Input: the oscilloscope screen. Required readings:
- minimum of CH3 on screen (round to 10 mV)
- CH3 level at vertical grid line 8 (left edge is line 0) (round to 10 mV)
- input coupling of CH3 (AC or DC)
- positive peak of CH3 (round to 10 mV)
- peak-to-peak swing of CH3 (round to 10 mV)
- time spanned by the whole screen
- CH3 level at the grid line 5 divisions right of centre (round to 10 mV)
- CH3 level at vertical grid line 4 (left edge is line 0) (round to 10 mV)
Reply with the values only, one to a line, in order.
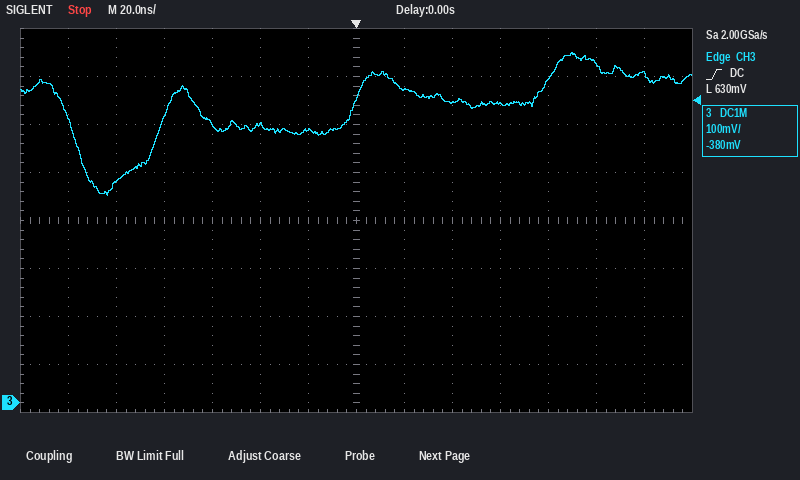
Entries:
430 mV
650 mV
DC
730 mV
300 mV
280 ns
710 mV
580 mV
